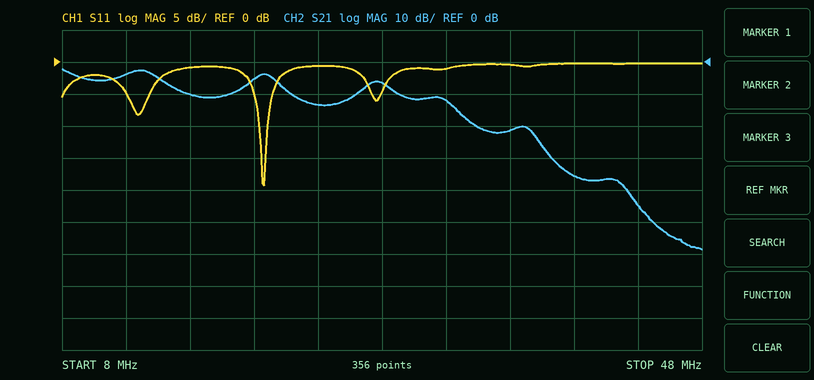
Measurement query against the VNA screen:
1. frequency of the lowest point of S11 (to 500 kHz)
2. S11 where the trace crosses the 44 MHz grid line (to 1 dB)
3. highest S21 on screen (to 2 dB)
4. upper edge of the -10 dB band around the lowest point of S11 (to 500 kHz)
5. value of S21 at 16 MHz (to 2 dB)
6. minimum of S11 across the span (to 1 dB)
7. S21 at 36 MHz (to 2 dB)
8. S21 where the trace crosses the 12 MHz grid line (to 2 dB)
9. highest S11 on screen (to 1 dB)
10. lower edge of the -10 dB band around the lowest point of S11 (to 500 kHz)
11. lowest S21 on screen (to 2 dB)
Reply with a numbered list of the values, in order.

1. 20.5 MHz
2. 0 dB
3. -2 dB
4. 21.0 MHz
5. -10 dB
6. -19 dB
7. -22 dB
8. -4 dB
9. 0 dB
10. 20.5 MHz
11. -58 dB
